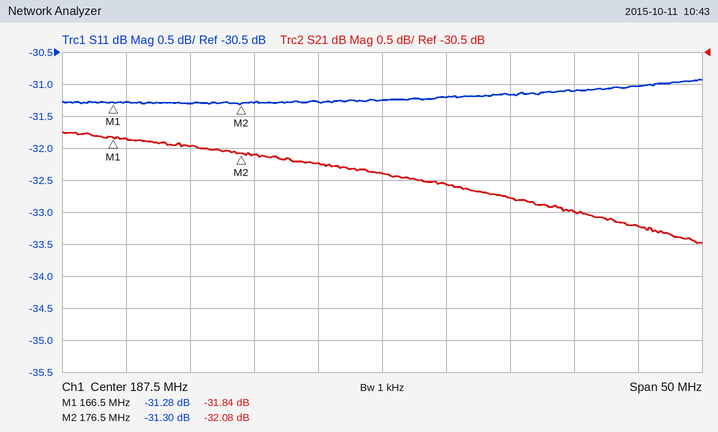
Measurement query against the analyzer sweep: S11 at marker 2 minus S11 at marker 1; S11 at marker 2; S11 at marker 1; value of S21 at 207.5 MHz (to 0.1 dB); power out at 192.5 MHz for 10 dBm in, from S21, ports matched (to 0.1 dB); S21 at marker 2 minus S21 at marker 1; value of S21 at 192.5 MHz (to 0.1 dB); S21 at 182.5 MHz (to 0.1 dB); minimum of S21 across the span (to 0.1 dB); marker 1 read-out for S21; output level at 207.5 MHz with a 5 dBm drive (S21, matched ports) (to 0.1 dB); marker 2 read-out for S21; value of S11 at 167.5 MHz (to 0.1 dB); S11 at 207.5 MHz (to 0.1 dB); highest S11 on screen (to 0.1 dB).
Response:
-0.02 dB
-31.30 dB
-31.28 dB
-33.2 dB
-22.6 dBm
-0.24 dB
-32.6 dB
-32.2 dB
-33.5 dB
-31.84 dB
-28.2 dBm
-32.08 dB
-31.3 dB
-31.0 dB
-30.9 dB
